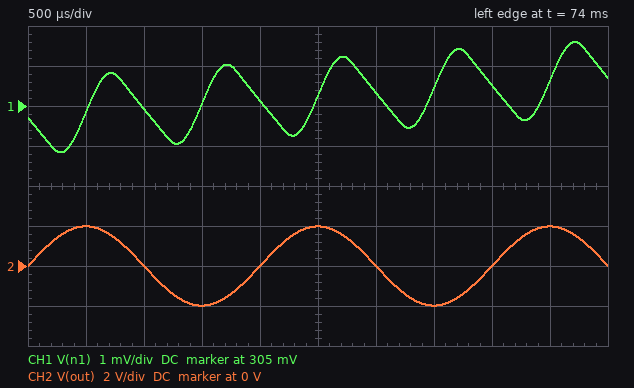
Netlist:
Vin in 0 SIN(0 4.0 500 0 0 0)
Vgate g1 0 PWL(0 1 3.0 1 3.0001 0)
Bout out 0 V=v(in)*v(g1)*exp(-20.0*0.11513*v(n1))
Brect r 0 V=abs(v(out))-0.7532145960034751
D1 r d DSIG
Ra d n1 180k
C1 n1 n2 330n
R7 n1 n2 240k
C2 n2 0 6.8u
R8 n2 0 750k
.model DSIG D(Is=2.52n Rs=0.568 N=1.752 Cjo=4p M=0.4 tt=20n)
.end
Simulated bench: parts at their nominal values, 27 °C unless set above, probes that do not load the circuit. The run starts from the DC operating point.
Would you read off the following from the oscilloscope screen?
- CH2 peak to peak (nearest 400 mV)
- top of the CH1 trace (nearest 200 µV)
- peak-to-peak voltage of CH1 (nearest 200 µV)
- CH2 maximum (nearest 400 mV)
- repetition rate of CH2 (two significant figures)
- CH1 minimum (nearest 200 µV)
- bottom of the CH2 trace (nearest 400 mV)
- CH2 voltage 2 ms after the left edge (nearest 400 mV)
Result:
4.0 V
306.6 mV
2.8 mV
2.0 V
500 Hz
303.8 mV
-2.0 V
0 V
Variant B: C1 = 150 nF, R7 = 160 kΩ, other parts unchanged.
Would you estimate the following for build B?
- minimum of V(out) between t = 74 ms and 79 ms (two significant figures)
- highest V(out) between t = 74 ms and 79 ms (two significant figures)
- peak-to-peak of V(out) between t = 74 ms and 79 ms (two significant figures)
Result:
-2.1 V
2.1 V
4.2 V
